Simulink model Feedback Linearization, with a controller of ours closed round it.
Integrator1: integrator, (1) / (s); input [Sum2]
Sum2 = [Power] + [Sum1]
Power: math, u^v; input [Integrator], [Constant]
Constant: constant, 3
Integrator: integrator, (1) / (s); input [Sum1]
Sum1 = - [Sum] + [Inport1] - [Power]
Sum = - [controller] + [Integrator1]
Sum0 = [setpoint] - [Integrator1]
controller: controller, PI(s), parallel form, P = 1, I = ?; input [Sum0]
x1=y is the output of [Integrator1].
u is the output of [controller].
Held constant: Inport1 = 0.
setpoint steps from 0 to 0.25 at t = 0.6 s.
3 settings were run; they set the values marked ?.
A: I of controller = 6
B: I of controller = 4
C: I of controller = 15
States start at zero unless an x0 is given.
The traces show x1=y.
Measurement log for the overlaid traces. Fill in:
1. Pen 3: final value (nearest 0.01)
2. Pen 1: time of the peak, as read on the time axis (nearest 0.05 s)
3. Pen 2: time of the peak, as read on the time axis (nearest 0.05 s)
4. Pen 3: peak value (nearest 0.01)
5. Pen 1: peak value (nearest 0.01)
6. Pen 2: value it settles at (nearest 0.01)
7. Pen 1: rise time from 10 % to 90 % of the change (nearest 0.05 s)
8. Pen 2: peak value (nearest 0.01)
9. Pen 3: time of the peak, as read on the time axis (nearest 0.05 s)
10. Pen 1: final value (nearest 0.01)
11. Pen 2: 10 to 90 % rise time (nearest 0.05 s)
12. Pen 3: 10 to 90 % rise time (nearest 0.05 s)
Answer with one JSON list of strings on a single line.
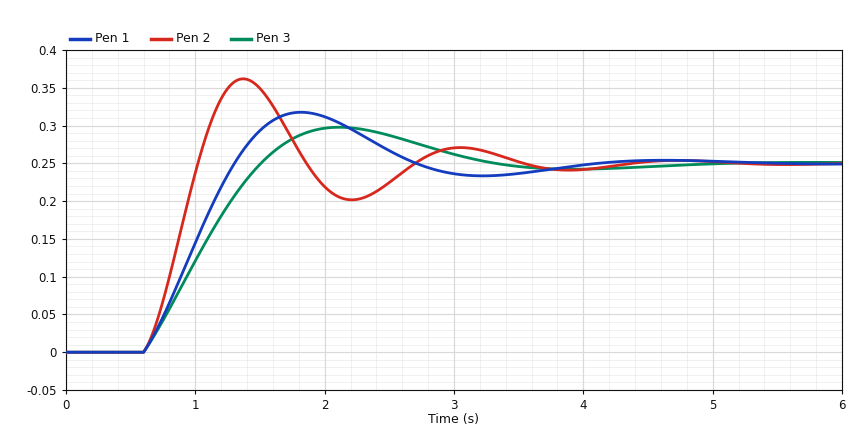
["0.25", "1.80 s", "1.35 s", "0.30", "0.32", "0.25", "0.55 s", "0.36", "2.10 s", "0.25", "0.30 s", "0.70 s"]
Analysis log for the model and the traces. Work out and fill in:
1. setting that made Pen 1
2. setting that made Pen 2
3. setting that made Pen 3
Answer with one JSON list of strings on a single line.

["A", "C", "B"]
